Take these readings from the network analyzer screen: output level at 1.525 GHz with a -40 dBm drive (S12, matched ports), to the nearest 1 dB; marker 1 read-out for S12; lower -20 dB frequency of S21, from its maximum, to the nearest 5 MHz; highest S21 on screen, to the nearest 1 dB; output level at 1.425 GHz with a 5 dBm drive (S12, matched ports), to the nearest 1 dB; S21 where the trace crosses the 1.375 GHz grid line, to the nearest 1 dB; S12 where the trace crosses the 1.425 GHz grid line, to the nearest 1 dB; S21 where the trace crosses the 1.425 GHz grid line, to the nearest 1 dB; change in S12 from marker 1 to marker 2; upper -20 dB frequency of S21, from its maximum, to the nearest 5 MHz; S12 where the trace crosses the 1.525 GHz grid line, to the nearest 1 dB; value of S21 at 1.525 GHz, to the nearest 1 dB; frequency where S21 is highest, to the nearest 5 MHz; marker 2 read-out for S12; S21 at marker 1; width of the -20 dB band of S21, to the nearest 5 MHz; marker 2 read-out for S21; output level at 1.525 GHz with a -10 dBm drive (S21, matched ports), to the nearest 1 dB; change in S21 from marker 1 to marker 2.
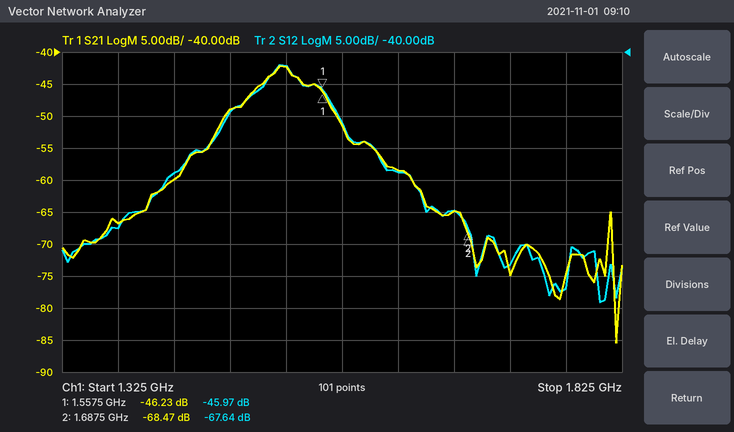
-82 dBm
-45.97 dB
1.405 GHz
-42 dB
-54 dBm
-67 dB
-59 dB
-60 dB
-21.67 dB
1.645 GHz
-42 dB
-42 dB
1.520 GHz
-67.64 dB
-46.23 dB
240 MHz
-68.47 dB
-52 dBm
-22.24 dB
